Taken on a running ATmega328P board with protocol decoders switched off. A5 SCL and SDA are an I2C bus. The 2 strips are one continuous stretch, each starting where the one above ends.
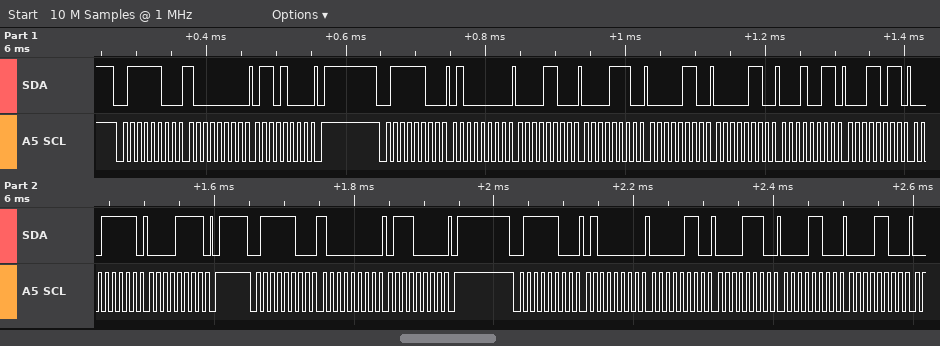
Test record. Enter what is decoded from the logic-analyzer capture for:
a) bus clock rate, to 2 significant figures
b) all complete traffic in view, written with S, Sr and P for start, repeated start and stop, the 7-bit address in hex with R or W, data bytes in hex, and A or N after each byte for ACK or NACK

100 kHz
S 3EW A 80 A 68 A P S 3EW A 40 A 0C A 0E A 06 A 06 A 13 A 1B A 1F A 0F A P S 3EW A 80 A 70 A P S 3EW A 40 A 06 A 0E A 0C A 0C A
